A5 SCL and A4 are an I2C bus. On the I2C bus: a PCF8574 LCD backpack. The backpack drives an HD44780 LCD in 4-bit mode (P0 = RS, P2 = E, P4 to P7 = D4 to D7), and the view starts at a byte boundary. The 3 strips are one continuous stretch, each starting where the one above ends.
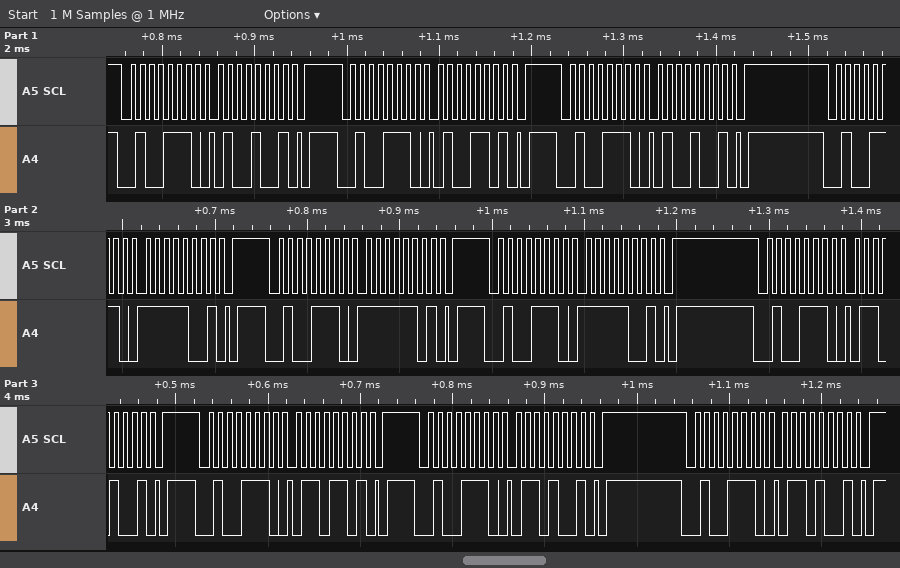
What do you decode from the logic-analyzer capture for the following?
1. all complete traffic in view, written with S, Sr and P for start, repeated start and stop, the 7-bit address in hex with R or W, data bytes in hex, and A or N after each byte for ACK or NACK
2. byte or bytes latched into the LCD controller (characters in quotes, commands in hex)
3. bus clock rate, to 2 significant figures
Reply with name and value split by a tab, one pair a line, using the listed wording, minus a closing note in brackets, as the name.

all complete traffic in view, written with S, Sr and P for start, repeated start and stop, the 7-bit address in hex with R or W, data bytes in hex, and A or N after each byte for ACK or NACK	S 27W A 49 A P S 27W A 4D A P S 27W A 49 A P S 27W A F9 A P S 27W A FD A P S 27W A F9 A P S 27W A 69 A P S 27W A 6D A P S 27W A 69 A P S 27W A 69 A P
byte or bytes latched into the LCD controller	'O'
bus clock rate, to 2 significant figures	100 kHz
